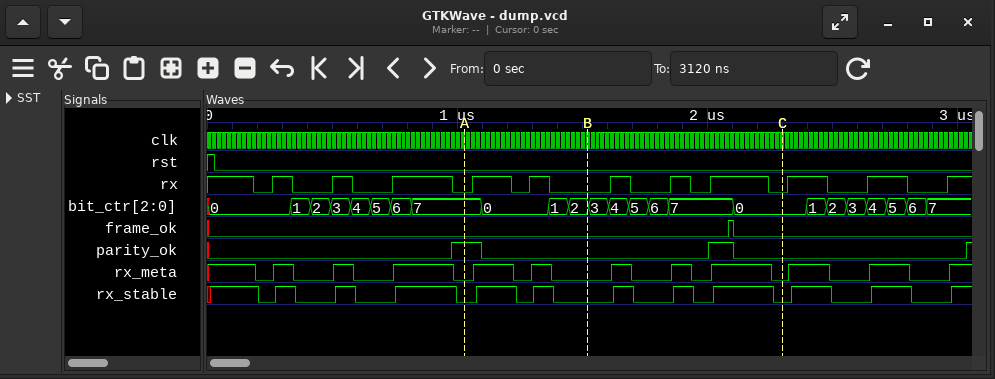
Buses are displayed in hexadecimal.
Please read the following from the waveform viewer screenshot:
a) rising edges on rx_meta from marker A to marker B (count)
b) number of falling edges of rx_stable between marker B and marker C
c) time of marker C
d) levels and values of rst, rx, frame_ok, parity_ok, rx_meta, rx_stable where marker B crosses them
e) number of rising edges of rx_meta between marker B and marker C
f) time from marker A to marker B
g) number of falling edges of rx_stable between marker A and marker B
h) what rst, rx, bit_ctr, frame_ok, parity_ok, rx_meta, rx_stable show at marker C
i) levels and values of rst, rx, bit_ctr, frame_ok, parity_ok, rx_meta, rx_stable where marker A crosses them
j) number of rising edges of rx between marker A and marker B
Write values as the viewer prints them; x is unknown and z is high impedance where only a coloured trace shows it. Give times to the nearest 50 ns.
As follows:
2
3
2300 ns
rst=0, rx=0, frame_ok=0, parity_ok=0, rx_meta=0, rx_stable=0
3
500 ns
2
rst=0, rx=0, bit_ctr=0, frame_ok=0, parity_ok=0, rx_meta=0, rx_stable=0
rst=0, rx=0, bit_ctr=7, frame_ok=0, parity_ok=1, rx_meta=0, rx_stable=0
2
